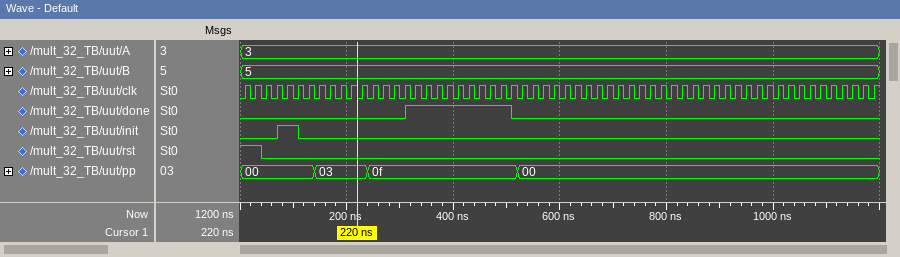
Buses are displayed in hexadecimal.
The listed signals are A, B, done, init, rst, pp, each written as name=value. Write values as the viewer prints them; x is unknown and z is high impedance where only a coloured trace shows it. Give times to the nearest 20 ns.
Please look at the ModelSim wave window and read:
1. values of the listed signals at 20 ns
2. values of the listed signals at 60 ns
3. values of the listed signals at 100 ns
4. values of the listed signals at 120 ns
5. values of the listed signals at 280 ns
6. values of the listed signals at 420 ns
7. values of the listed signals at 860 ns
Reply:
A=3, B=5, done=0, init=0, rst=1, pp=00
A=3, B=5, done=0, init=0, rst=0, pp=00
A=3, B=5, done=0, init=1, rst=0, pp=00
A=3, B=5, done=0, init=0, rst=0, pp=00
A=3, B=5, done=0, init=0, rst=0, pp=0f
A=3, B=5, done=1, init=0, rst=0, pp=0f
A=3, B=5, done=0, init=0, rst=0, pp=00
